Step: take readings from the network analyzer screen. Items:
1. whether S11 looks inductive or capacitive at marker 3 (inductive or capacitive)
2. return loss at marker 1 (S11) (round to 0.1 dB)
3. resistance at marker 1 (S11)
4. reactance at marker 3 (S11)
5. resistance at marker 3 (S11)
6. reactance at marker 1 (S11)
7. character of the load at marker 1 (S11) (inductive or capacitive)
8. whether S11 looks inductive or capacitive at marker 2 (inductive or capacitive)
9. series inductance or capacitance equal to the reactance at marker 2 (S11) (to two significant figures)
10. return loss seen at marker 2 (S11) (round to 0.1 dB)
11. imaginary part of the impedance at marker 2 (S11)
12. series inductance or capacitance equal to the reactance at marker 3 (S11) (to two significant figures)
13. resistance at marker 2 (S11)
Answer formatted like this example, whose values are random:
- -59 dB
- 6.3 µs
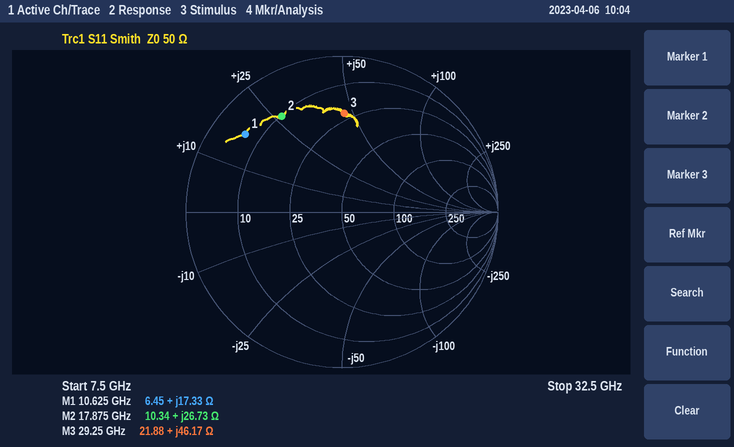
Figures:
- inductive
- 2.0 dB
- 6.45 Ω
- +46.17 Ω
- 21.88 Ω
- +17.33 Ω
- inductive
- inductive
- 240 pH
- 2.8 dB
- +26.73 Ω
- 250 pH
- 10.34 Ω
